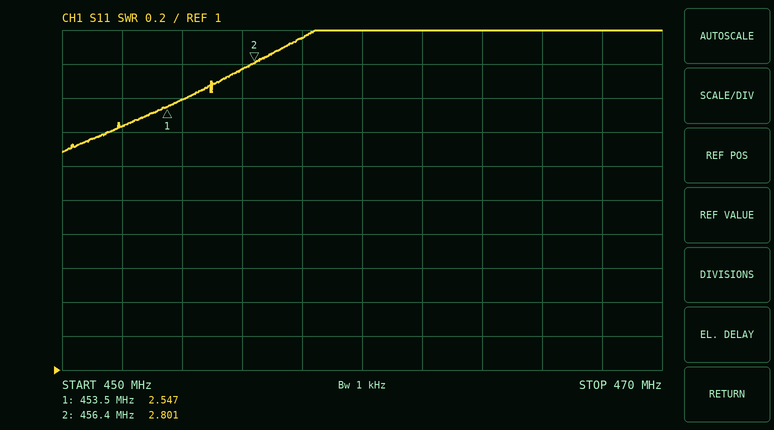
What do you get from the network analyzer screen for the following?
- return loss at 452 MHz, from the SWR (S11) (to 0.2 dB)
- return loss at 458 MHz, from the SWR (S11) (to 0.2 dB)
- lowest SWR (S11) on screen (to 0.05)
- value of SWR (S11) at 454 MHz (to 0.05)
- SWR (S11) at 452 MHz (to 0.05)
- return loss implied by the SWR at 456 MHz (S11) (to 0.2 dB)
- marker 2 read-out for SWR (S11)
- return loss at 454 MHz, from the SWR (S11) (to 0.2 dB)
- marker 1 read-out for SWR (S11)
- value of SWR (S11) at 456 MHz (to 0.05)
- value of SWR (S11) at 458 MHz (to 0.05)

7.6 dB
6.2 dB
2.30
2.60
2.45
6.6 dB
2.801
7.0 dB
2.547
2.75
2.95
